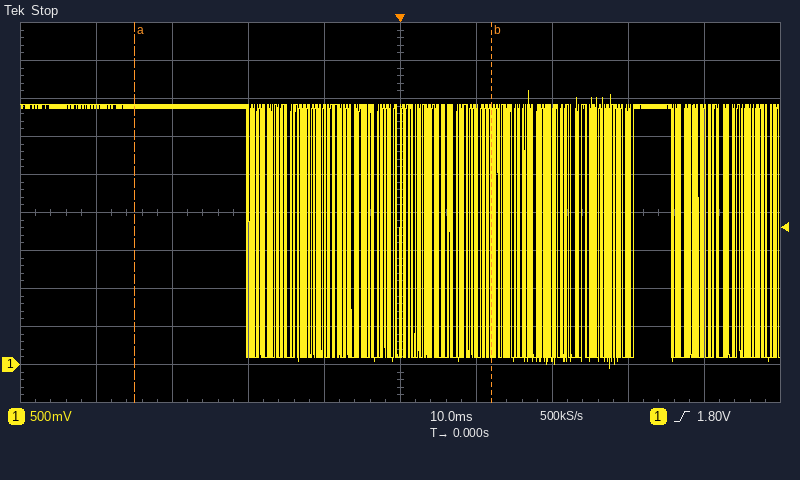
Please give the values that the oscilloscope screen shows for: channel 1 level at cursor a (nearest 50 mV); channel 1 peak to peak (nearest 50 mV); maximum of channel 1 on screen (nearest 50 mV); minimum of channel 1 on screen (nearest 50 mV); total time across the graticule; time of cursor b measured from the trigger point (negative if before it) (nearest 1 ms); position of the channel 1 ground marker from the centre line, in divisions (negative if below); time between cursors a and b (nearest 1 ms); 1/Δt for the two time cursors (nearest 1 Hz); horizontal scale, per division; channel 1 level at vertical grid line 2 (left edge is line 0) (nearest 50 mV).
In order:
3.40 V
3.65 V
3.60 V
-50 mV
100 ms
+12 ms
-4.0 div
47 ms
21 Hz
10 ms
3.40 V
